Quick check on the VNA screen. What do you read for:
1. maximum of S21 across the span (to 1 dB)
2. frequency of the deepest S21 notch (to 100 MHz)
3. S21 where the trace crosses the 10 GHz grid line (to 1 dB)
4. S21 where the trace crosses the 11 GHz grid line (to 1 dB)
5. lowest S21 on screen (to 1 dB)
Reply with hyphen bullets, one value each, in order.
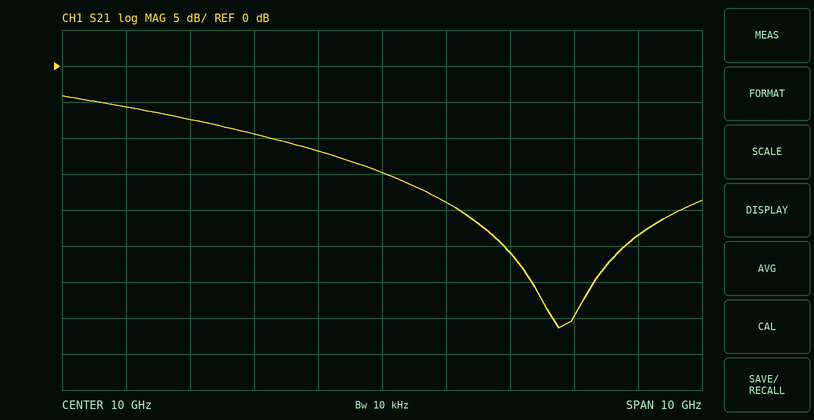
- -4 dB
- 12.8 GHz
- -15 dB
- -19 dB
- -36 dB
